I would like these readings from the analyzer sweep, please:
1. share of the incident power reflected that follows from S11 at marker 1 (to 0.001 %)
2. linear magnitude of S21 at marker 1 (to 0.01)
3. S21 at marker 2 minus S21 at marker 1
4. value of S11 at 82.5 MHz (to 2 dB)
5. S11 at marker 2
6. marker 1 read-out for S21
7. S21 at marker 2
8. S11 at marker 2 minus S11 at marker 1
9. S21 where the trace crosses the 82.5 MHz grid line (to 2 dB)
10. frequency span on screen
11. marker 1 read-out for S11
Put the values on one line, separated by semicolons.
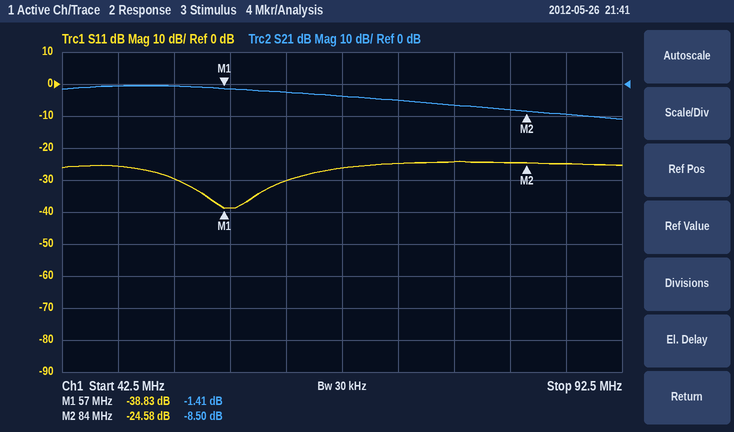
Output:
0.013 %; 0.85; -7.09 dB; -24 dB; -24.58 dB; -1.41 dB; -8.50 dB; 14.25 dB; -8 dB; 50 MHz; -38.83 dB
